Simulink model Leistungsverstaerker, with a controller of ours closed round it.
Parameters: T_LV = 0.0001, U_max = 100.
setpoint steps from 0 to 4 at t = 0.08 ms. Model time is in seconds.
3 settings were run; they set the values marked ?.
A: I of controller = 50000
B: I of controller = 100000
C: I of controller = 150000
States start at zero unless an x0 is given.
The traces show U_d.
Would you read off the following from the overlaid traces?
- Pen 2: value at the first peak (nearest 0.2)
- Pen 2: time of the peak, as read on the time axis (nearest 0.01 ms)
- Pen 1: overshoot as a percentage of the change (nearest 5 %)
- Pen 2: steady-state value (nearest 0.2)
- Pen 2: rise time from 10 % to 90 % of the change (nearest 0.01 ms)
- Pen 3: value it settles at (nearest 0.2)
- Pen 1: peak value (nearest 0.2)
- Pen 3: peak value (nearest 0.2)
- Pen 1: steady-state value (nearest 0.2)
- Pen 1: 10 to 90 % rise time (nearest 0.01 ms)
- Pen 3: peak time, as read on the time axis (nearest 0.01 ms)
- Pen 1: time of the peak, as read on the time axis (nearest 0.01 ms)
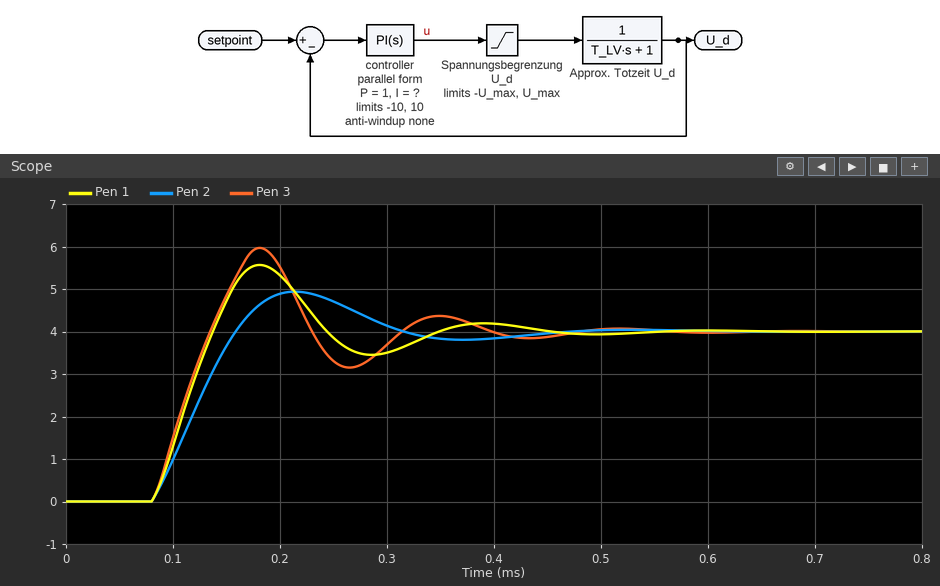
5.0
0.21 ms
40 %
4.0
0.06 ms
4.0
5.6
6.0
4.0
0.04 ms
0.18 ms
0.18 ms
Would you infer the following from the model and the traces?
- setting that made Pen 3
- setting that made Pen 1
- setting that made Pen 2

C
B
A
